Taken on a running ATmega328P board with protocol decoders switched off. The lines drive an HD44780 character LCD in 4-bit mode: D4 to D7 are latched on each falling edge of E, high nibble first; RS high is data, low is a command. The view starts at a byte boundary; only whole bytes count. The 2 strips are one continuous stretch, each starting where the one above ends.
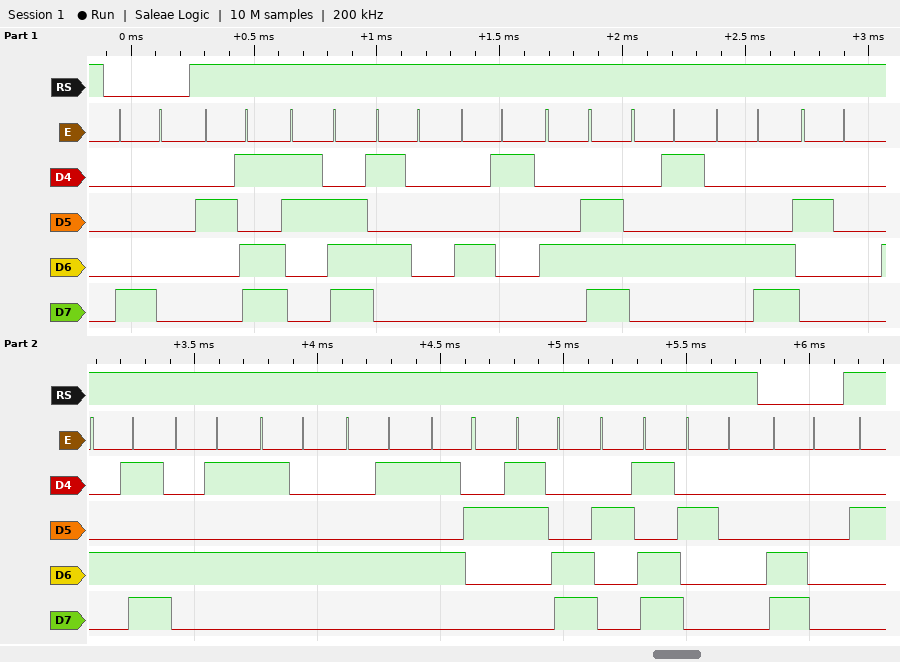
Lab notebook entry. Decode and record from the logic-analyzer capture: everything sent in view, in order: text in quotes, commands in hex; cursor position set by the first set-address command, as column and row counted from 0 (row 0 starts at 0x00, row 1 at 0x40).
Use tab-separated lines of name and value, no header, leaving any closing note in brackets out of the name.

everything sent in view, in order: text in quotes, commands in hex	0x80 "->PANEL METER<- " 0xC0
cursor position set by the first set-address command, as column and row counted from 0	column 0, row 0
